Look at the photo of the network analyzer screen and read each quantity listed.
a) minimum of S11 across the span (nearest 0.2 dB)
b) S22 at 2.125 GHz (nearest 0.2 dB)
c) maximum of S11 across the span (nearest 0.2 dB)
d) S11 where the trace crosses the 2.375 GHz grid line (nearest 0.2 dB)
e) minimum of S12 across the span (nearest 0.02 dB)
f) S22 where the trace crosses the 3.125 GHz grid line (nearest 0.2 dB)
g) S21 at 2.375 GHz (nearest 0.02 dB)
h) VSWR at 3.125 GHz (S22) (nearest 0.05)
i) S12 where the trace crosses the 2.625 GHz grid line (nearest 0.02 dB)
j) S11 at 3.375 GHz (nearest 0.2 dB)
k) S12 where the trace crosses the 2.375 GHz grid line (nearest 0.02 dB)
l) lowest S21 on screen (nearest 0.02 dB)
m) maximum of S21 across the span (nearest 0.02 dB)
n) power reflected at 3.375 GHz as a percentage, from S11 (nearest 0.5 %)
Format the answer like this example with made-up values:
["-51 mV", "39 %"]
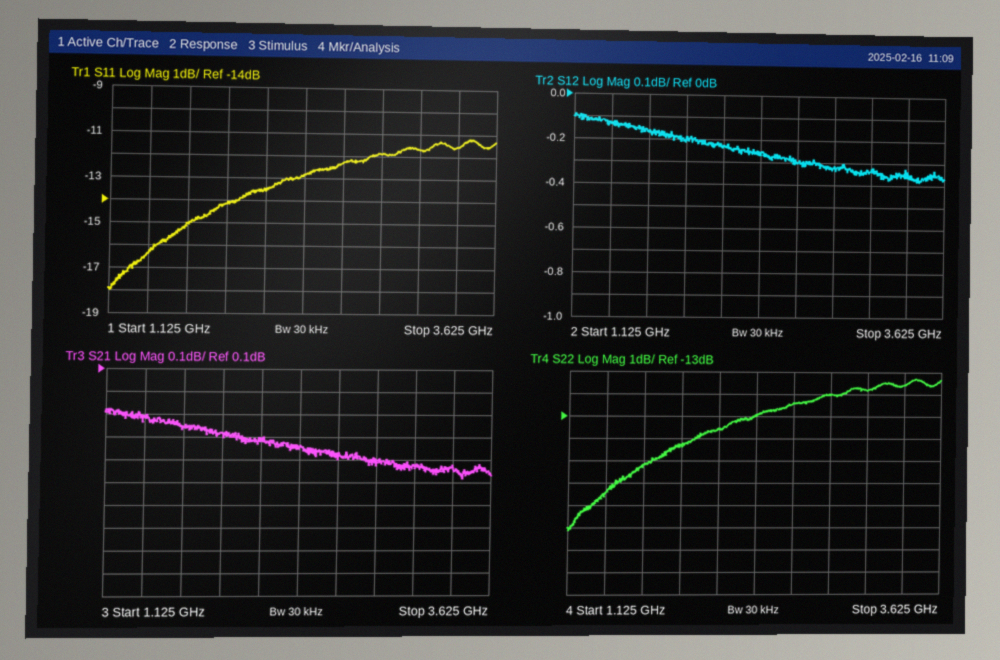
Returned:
["-18.0 dB", "-13.6 dB", "-11.2 dB", "-12.8 dB", "-0.38 dB", "-11.8 dB", "-0.24 dB", "1.70", "-0.30 dB", "-11.6 dB", "-0.26 dB", "-0.38 dB", "-0.08 dB", "7.0 %"]
